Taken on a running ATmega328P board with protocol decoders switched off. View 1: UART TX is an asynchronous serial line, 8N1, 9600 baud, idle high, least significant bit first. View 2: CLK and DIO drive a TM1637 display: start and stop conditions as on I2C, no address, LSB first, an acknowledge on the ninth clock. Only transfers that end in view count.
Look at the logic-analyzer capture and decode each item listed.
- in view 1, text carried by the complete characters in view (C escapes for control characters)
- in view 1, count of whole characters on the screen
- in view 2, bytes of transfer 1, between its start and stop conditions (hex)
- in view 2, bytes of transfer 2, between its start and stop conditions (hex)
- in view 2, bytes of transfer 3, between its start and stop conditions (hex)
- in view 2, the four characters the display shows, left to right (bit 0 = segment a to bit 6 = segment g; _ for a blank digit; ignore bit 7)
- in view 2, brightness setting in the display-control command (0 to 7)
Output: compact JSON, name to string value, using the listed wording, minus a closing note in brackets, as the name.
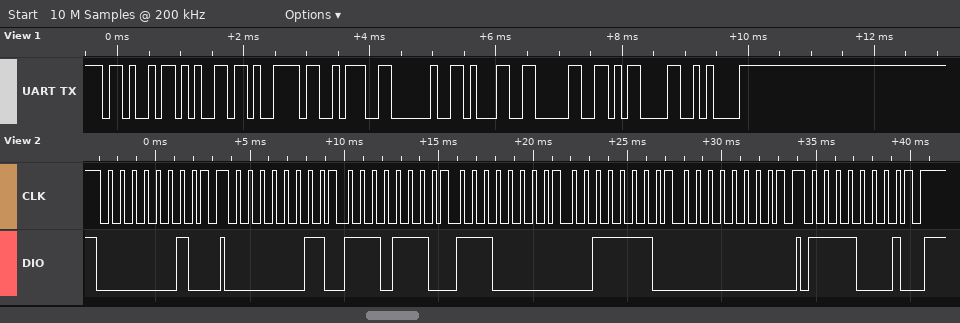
{"in view 1, text carried by the complete characters in view": "\"Key: 10\\r\\n\"", "in view 1, count of whole characters on the screen": "9", "in view 2, bytes of transfer 1, between its start and stop conditions": "40", "in view 2, bytes of transfer 2, between its start and stop conditions": "C0 77 07 7C 00", "in view 2, bytes of transfer 3, between its start and stop conditions": "8F", "in view 2, the four characters the display shows, left to right": "A7b_", "in view 2, brightness setting in the display-control command": "7"}
